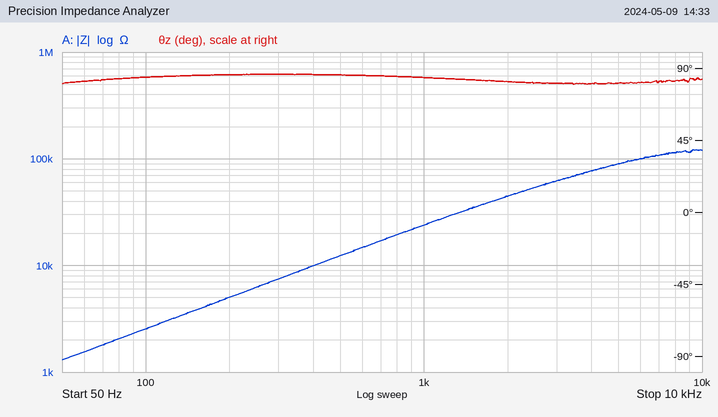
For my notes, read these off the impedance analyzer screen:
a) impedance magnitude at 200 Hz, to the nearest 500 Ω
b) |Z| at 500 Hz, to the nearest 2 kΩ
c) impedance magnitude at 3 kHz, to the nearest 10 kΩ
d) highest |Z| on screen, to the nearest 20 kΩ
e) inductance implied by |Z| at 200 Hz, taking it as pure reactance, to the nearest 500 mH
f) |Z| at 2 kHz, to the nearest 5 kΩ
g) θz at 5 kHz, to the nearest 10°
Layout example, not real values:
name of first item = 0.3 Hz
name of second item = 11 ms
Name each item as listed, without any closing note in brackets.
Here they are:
impedance magnitude at 200 Hz, to the nearest 500 Ω = 5.0 kΩ
|Z| at 500 Hz, to the nearest 2 kΩ = 12 kΩ
impedance magnitude at 3 kHz, to the nearest 10 kΩ = 60 kΩ
highest |Z| on screen, to the nearest 20 kΩ = 120 kΩ
inductance implied by |Z| at 200 Hz, taking it as pure reactance, to the nearest 500 mH = 4.0 H
|Z| at 2 kHz, to the nearest 5 kΩ = 45 kΩ
θz at 5 kHz, to the nearest 10° = 80°
